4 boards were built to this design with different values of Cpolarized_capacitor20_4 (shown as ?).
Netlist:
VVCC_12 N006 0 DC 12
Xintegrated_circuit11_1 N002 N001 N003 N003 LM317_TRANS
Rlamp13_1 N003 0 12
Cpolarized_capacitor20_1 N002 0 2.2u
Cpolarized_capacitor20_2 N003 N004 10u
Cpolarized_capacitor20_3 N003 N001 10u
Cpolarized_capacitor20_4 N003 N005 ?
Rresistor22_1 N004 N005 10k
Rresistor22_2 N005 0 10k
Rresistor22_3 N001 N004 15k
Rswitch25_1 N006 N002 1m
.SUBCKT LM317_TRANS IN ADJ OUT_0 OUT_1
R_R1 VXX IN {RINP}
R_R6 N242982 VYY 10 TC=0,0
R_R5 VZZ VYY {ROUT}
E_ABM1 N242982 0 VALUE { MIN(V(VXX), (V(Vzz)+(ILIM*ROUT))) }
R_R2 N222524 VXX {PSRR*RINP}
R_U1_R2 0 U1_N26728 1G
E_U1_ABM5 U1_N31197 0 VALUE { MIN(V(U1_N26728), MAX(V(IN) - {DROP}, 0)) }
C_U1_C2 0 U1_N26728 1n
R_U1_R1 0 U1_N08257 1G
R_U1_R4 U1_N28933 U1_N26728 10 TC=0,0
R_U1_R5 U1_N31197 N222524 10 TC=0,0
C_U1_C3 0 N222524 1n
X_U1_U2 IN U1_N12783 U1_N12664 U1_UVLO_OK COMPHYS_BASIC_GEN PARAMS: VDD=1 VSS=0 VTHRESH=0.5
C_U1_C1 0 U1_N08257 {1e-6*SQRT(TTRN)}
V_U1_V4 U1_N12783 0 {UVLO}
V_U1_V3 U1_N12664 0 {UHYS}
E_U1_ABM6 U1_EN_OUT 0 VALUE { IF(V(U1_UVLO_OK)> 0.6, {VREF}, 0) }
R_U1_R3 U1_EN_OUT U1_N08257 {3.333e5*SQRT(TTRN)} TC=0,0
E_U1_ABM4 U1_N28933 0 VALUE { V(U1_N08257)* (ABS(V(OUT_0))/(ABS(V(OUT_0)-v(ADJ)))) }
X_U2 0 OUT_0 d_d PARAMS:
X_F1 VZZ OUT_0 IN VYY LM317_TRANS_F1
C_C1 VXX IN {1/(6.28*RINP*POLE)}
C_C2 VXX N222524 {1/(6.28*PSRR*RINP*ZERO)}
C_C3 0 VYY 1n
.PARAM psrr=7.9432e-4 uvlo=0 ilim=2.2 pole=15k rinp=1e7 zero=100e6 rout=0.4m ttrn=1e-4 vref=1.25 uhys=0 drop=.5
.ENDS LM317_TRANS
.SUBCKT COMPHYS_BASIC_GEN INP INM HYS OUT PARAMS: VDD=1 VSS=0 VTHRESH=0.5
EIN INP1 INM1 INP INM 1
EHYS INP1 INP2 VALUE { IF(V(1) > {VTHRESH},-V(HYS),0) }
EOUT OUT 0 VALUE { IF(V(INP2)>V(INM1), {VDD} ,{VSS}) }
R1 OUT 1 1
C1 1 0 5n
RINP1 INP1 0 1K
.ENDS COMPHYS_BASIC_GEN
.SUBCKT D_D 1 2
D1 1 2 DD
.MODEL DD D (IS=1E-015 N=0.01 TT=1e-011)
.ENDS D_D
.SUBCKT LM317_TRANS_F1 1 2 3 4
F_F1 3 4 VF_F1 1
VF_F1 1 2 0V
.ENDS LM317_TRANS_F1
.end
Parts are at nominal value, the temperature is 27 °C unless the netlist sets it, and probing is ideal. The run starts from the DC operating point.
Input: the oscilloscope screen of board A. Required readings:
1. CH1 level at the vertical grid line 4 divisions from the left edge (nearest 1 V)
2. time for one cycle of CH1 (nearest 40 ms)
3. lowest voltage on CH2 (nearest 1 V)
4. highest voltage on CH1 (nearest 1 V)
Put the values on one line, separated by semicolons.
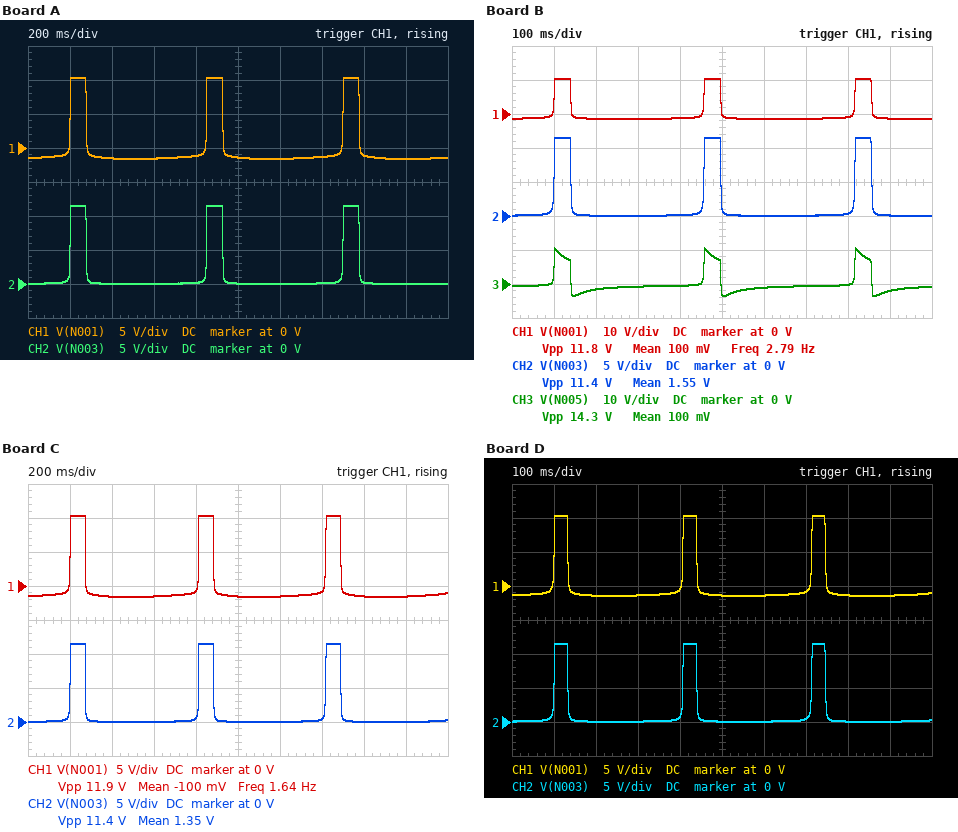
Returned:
-1 V; 640 ms; 0 V; 10 V
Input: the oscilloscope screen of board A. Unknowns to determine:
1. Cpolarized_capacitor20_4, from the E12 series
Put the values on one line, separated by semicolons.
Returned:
33 µF
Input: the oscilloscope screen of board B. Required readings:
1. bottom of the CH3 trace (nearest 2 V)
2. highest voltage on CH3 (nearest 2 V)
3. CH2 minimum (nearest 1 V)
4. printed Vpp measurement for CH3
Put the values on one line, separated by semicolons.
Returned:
-4 V; 10 V; 0 V; 14.3 V
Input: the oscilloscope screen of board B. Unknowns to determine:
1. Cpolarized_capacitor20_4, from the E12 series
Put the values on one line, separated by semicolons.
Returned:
6.8 µF
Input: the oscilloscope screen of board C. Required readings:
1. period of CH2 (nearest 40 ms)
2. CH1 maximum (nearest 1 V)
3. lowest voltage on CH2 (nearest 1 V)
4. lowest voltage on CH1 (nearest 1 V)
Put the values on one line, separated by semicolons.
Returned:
600 ms; 10 V; 0 V; -2 V
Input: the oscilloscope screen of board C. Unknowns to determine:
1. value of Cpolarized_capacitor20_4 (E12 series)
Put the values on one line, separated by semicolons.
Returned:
27 µF
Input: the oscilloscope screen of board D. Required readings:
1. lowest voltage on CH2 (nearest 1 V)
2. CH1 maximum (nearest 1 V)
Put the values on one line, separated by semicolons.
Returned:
0 V; 10 V
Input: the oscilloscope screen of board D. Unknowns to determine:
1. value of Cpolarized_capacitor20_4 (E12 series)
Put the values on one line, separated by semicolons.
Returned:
4.7 µF
